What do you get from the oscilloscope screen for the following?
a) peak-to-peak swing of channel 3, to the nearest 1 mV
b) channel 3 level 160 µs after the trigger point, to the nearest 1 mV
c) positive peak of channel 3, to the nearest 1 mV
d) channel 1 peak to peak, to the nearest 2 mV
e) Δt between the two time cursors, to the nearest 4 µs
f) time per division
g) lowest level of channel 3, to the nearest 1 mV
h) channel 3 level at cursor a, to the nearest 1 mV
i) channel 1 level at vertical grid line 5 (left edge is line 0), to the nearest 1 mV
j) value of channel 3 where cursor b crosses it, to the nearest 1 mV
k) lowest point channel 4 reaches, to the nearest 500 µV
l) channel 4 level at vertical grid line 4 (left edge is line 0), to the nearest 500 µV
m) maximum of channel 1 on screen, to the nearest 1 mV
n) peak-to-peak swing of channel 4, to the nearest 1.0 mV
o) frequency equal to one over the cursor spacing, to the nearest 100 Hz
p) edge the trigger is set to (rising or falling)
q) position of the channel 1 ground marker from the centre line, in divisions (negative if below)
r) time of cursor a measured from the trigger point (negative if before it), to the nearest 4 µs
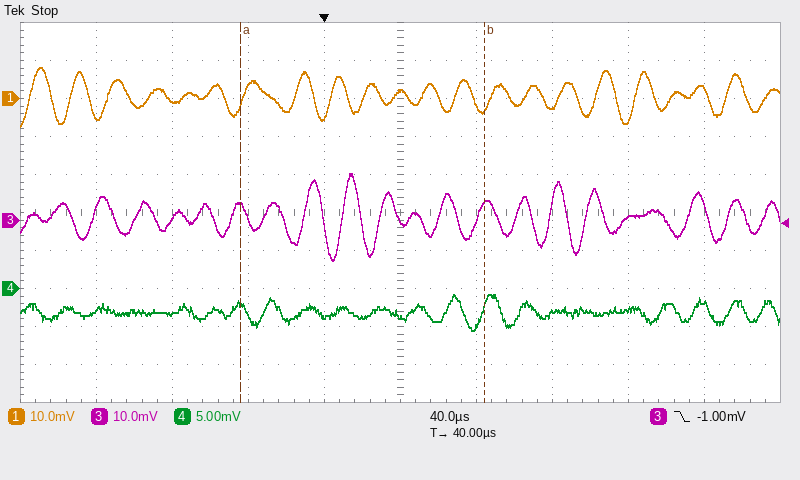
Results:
23 mV
1 mV
12 mV
16 mV
128 µs
40 µs
-11 mV
4 mV
2 mV
4 mV
-5.5 mV
-3.5 mV
8 mV
5.0 mV
7.8 kHz
falling
+3.0 div
-44 µs
